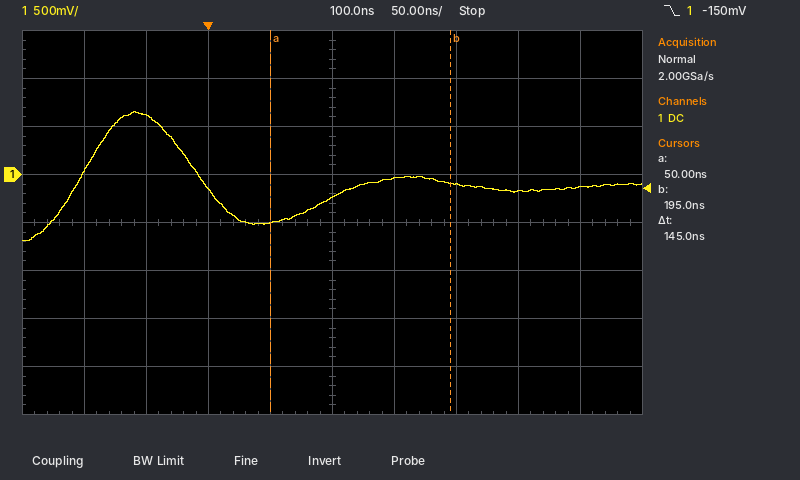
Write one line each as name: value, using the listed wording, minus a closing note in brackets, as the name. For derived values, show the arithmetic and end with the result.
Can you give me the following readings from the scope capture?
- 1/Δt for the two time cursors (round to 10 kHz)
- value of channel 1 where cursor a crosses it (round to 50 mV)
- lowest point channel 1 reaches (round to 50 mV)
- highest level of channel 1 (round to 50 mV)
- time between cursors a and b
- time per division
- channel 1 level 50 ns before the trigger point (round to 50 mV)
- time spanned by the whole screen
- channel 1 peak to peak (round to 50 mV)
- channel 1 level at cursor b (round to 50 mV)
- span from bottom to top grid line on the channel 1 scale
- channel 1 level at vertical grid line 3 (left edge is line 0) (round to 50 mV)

1/Δt for the two time cursors: 1 / 145 ns ≈ 6.90 MHz
value of channel 1 where cursor a crosses it: -500 mV
lowest point channel 1 reaches: -700 mV
highest level of channel 1: 650 mV
time between cursors a and b: 145 ns
time per division: 50 ns
channel 1 level 50 ns before the trigger point: 600 mV
time spanned by the whole screen: 500 ns
channel 1 peak to peak: 650 mV − (-700 mV) = 1.35 V
channel 1 level at cursor b: -100 mV
span from bottom to top grid line on the channel 1 scale: 4 V
channel 1 level at vertical grid line 3 (left edge is line 0): -150 mV
